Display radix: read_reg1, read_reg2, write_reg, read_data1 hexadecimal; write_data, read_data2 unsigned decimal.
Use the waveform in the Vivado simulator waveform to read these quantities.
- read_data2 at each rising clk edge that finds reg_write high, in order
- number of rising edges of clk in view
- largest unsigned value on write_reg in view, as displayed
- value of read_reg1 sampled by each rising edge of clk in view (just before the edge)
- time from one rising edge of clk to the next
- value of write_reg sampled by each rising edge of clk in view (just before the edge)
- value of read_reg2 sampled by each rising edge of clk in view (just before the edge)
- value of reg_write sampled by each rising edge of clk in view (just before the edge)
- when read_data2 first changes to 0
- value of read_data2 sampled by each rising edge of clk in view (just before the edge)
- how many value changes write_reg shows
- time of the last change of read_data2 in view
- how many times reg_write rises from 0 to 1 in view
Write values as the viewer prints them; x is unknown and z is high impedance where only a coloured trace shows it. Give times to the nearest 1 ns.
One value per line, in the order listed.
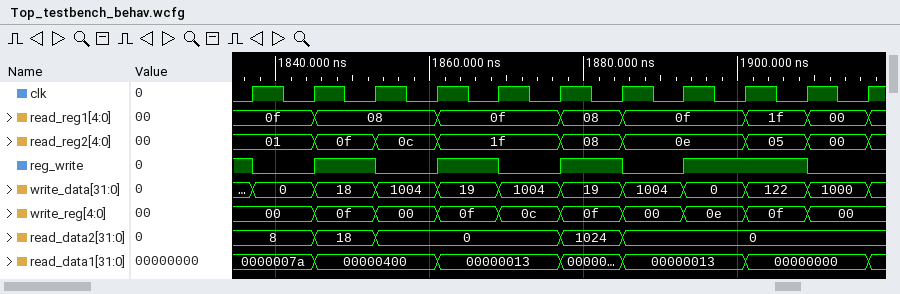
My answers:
8, 18, 0, 1024, 0, 0
11
0f
0f, 0f, 08, 08, 0f, 0f, 08, 0f, 0f, 1f, 00
8 ns
00, 00, 0f, 00, 0f, 0c, 0f, 00, 0e, 0f, 00
01, 01, 0f, 0c, 1f, 1f, 08, 0e, 0e, 05, 00
1 0 1 0 1 0 1 0 1 1 0
1853 ns
8, 8, 18, 0, 0, 0, 1024, 0, 0, 0, 0
9
1885 ns
4
